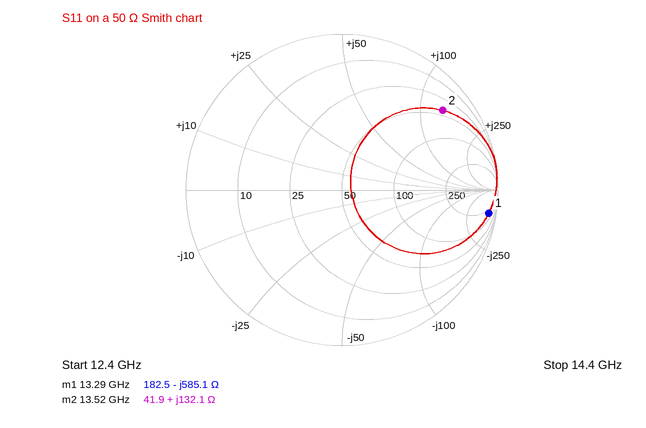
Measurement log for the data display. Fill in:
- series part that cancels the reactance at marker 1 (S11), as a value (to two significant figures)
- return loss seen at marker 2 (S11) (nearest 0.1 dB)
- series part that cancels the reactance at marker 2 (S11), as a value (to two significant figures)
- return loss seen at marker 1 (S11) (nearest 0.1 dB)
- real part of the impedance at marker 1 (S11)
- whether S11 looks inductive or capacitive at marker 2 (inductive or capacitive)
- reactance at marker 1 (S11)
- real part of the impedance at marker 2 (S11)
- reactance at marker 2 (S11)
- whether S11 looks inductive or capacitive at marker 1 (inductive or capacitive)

7.0 nH
1.7 dB
89 fF
0.4 dB
182.5 Ω
inductive
-585.1 Ω
41.9 Ω
+132.1 Ω
capacitive
